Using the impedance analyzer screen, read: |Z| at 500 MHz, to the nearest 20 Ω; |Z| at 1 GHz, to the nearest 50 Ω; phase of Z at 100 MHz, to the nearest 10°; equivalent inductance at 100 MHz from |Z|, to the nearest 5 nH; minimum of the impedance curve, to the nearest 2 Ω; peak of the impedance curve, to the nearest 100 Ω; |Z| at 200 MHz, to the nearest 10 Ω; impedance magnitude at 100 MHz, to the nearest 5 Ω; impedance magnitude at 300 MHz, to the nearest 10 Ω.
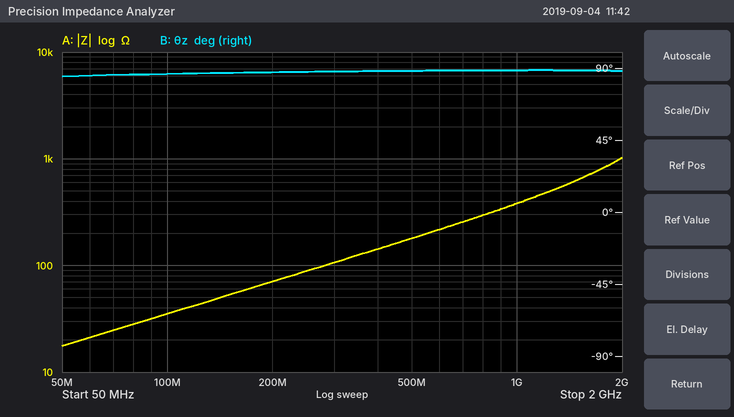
180 Ω
400 Ω
90°
55 nH
18 Ω
1.0 kΩ
70 Ω
35 Ω
110 Ω
